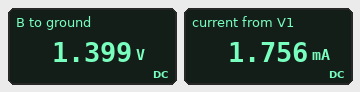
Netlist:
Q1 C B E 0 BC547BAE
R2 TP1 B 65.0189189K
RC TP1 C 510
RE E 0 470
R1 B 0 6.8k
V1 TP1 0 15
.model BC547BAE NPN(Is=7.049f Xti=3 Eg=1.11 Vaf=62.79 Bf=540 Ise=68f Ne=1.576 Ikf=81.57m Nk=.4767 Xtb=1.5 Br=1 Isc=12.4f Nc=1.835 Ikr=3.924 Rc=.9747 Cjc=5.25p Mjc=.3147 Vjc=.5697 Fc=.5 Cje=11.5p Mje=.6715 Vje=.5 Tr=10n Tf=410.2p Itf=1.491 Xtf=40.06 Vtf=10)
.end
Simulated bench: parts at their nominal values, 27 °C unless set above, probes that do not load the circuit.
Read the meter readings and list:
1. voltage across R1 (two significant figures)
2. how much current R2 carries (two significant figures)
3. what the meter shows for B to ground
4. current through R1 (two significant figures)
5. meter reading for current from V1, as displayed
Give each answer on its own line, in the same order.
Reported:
1.4 V
210 µA
1.399 V
210 µA
1.756 mA
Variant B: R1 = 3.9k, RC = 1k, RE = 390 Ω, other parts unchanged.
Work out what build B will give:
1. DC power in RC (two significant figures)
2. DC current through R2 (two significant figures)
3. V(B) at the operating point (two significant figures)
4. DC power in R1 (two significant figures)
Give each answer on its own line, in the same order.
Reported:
270 µW
220 µA
840 mV
180 µW
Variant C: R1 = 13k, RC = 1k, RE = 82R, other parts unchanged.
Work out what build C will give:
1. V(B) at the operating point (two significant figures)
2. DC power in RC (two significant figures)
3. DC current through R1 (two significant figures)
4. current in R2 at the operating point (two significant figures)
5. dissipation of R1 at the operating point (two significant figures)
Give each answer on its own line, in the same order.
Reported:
1.9 V
190 mW
140 µA
200 µA
270 µW
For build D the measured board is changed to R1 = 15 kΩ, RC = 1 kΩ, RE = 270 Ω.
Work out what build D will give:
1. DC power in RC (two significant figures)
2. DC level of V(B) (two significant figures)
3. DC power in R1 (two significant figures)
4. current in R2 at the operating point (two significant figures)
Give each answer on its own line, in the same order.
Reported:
50 mW
2.6 V
460 µW
190 µA
